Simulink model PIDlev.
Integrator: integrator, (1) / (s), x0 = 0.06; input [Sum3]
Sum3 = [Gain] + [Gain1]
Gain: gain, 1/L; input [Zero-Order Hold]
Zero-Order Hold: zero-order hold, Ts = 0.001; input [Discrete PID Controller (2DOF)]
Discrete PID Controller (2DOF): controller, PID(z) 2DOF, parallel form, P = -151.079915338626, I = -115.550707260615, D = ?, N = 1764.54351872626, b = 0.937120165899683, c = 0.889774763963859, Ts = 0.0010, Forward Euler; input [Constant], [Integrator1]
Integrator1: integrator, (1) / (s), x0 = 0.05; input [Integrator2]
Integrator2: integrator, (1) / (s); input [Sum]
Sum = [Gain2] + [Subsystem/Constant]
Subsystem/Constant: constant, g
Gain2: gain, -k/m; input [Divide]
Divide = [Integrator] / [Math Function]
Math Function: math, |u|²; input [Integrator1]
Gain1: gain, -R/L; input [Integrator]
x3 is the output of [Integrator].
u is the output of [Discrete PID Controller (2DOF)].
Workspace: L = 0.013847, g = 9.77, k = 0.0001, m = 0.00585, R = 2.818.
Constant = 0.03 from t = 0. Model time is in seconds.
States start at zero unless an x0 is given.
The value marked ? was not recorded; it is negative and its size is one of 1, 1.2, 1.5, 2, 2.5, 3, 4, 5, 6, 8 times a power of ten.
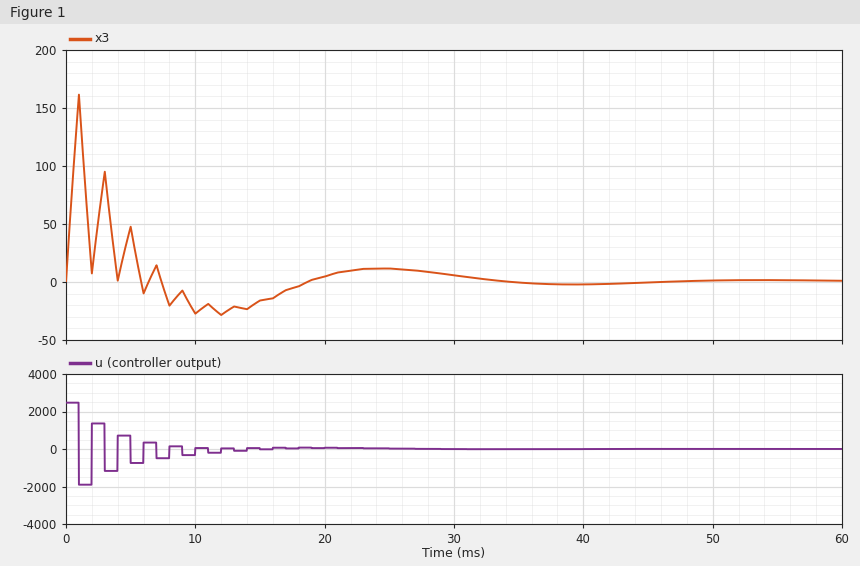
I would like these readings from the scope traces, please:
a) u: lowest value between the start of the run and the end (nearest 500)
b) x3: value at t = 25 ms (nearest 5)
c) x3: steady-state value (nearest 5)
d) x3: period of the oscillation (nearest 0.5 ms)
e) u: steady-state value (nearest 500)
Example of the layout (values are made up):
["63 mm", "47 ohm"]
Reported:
["-2000", "10", "0", "2.0 ms", "0"]
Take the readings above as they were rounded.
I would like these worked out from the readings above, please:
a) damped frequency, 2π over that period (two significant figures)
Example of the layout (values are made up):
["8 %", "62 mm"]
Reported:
["3.1 rad/ms"]
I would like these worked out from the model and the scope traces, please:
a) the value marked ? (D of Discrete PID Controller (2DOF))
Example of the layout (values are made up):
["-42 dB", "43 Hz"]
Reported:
["-60"]
